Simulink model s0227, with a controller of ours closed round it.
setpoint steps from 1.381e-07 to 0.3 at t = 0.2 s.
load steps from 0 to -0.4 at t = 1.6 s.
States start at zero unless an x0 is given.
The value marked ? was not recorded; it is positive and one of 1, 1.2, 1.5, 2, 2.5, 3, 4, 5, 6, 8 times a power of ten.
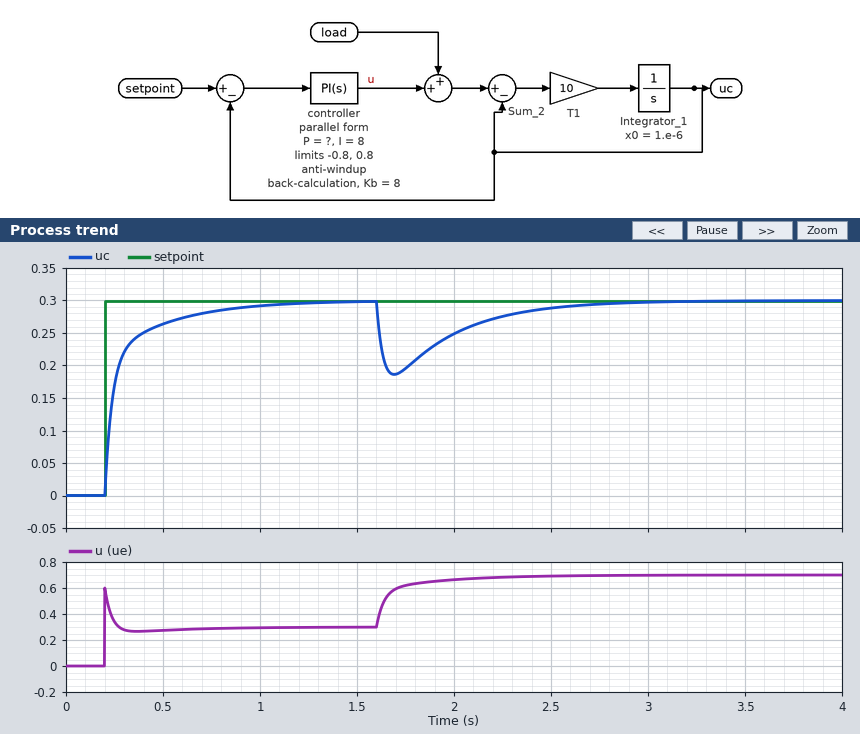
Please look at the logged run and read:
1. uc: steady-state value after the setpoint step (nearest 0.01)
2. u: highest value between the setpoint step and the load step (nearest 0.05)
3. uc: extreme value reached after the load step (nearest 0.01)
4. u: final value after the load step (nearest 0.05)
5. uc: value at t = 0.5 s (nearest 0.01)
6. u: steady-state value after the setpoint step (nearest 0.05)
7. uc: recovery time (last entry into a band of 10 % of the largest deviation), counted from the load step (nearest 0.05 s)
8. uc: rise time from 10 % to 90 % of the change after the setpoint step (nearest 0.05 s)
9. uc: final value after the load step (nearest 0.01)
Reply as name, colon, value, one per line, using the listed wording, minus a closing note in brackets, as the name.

uc: steady-state value after the setpoint step: 0.30
u: highest value between the setpoint step and the load step: 0.60
uc: extreme value reached after the load step: 0.19
u: final value after the load step: 0.70
uc: value at t = 0.5 s: 0.26
u: steady-state value after the setpoint step: 0.30
uc: recovery time (last entry into a band of 10 % of the largest deviation), counted from the load step: 0.90 s
uc: rise time from 10 % to 90 % of the change after the setpoint step: 0.35 s
uc: final value after the load step: 0.30
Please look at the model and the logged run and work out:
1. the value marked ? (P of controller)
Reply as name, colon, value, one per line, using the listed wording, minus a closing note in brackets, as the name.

the value marked ?: 2
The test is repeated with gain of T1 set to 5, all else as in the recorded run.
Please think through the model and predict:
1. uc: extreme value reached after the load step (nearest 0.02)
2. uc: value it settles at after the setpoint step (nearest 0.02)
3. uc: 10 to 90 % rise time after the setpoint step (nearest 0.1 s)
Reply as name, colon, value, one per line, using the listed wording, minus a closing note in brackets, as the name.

uc: extreme value reached after the load step: 0.20
uc: value it settles at after the setpoint step: 0.30
uc: 10 to 90 % rise time after the setpoint step: 0.3 s
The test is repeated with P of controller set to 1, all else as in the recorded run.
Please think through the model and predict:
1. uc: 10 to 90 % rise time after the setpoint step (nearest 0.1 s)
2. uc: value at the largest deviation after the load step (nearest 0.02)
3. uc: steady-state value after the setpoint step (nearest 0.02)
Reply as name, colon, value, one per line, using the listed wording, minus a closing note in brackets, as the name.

uc: 10 to 90 % rise time after the setpoint step: 0.3 s
uc: value at the largest deviation after the load step: 0.14
uc: steady-state value after the setpoint step: 0.30
